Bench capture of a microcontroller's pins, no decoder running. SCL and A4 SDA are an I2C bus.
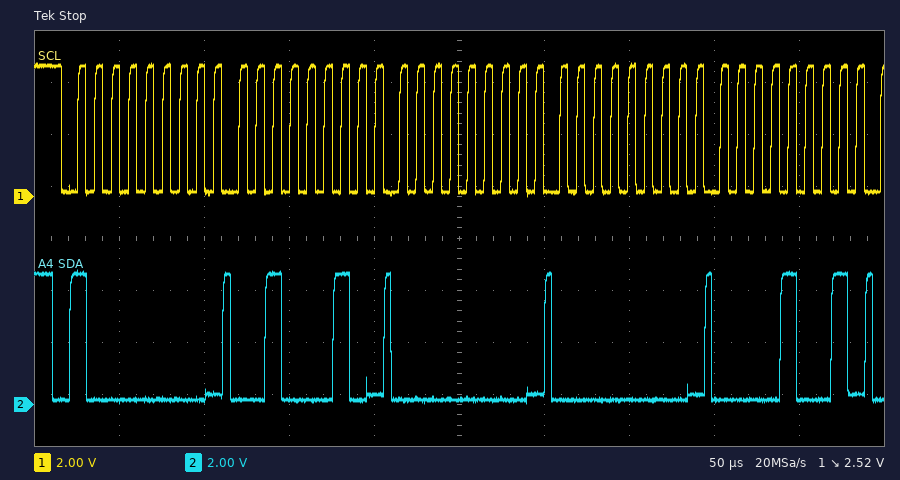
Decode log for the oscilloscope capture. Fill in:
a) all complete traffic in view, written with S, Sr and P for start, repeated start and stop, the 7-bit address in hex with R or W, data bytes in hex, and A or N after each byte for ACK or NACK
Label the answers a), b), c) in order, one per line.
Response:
a) S 40W A 22 A 00 A 00 A 09 A
